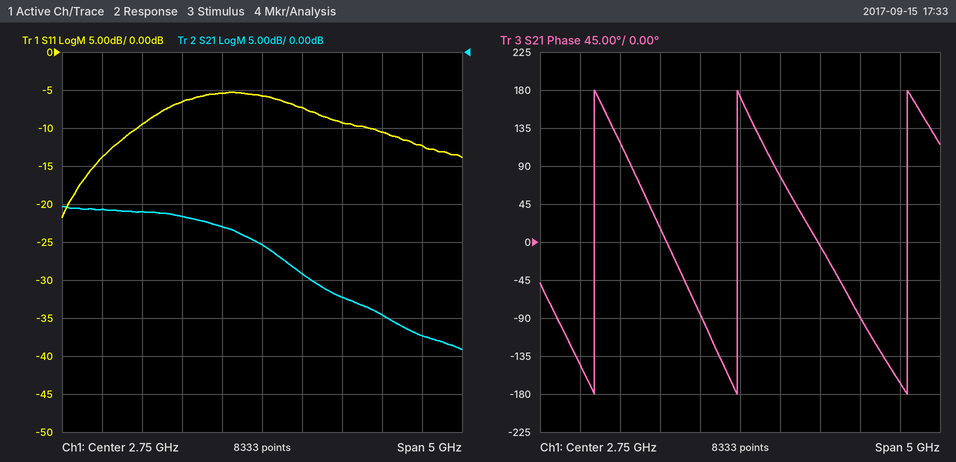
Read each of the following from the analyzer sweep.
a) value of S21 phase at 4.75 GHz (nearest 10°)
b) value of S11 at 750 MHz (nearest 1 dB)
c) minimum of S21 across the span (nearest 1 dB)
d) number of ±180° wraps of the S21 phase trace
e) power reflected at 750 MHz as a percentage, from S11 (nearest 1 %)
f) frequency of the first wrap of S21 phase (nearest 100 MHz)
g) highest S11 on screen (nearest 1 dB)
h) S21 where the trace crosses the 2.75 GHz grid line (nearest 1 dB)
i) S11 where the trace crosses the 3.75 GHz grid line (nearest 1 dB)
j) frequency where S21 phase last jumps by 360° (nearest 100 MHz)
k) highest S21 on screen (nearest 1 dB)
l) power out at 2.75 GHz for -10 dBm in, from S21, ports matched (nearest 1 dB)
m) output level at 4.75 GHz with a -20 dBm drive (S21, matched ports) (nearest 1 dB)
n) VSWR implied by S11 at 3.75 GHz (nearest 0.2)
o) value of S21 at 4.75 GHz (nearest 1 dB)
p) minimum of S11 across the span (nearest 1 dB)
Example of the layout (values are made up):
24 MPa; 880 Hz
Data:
-170°; -14 dB; -39 dB; 3; 4 %; 900 MHz; -5 dB; -25 dB; -9 dB; 4.8 GHz; -20 dB; -35 dBm; -57 dBm; 2.0; -37 dB; -22 dB
